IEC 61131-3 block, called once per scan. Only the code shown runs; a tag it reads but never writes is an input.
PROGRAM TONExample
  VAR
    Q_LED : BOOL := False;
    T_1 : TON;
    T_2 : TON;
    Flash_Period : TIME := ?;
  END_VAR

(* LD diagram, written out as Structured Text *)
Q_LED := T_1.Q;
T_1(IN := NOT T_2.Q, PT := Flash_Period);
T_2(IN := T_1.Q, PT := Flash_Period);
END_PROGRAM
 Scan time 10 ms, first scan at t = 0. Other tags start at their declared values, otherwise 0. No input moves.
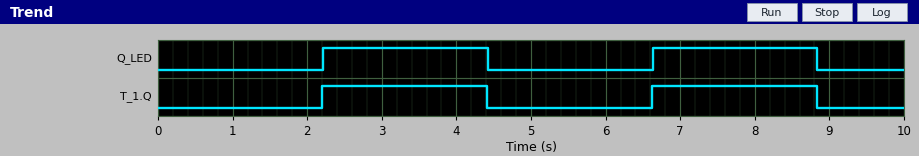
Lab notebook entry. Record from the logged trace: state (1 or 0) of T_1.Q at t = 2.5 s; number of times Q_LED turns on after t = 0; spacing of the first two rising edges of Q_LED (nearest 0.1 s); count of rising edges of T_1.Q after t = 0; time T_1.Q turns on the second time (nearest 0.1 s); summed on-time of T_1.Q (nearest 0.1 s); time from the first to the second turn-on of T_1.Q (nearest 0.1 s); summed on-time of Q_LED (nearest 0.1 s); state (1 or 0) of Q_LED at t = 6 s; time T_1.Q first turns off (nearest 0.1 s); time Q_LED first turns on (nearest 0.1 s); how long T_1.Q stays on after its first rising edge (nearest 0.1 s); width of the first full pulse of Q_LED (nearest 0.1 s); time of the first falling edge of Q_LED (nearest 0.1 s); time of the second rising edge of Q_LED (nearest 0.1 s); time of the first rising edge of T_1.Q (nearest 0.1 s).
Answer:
1
2
4.4 s
2
6.6 s
4.4 s
4.4 s
4.4 s
0
4.4 s
2.2 s
2.2 s
2.2 s
4.4 s
6.6 s
2.2 s
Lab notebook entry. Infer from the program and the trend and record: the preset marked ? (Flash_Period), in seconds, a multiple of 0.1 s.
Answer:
2.2 s
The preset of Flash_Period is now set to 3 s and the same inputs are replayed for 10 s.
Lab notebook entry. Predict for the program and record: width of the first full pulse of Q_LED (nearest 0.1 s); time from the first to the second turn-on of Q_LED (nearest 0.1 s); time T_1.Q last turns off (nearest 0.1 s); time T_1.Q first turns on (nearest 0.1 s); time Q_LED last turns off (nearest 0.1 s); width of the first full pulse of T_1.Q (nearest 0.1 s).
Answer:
3.0 s
6.0 s
6.0 s
3.0 s
6.0 s
3.0 s
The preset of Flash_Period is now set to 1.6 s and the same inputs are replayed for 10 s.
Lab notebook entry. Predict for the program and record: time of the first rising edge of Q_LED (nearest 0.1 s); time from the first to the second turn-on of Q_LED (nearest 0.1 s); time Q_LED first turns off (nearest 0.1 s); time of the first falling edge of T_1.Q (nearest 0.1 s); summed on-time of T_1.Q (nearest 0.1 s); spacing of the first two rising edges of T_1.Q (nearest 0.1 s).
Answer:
1.6 s
3.2 s
3.2 s
3.2 s
4.8 s
3.2 s
